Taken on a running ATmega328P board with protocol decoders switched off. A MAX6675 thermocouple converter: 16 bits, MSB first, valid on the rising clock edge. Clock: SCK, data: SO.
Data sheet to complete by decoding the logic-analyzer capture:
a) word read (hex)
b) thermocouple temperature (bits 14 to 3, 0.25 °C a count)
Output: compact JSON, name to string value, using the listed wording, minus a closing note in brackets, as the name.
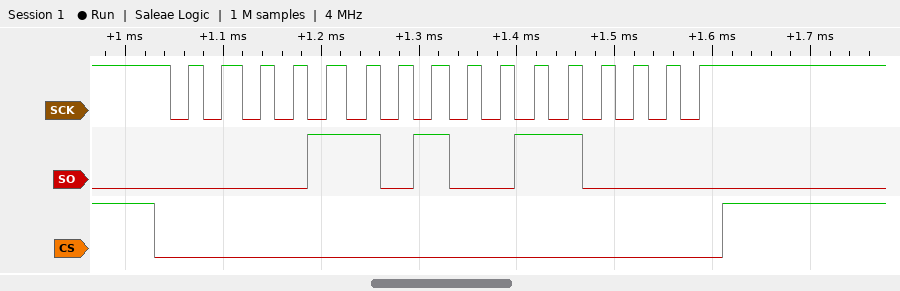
{"word read": "0x0D30", "thermocouple temperature": "105.50 °C"}
